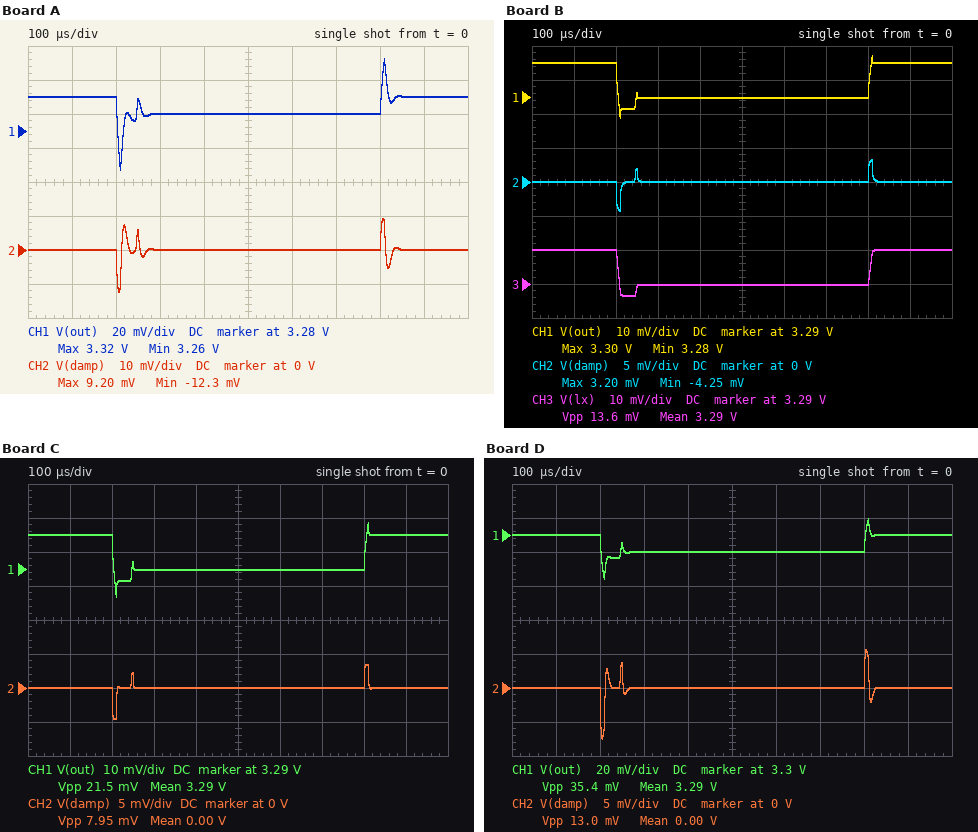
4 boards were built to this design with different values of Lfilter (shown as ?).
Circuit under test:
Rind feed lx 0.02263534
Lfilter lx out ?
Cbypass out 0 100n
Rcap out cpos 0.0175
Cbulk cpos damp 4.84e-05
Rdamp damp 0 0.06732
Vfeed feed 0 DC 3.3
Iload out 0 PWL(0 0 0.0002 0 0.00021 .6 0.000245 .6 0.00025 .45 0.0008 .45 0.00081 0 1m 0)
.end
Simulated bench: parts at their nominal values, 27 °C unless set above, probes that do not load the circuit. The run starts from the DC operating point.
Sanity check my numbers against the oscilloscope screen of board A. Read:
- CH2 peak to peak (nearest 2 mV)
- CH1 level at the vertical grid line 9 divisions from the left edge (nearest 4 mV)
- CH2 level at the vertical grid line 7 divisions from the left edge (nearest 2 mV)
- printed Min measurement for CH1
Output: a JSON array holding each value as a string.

["22 mV", "3.300 V", "0 V", "3.26 V"]
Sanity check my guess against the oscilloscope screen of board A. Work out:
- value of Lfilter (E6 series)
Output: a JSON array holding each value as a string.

["470 nH"]
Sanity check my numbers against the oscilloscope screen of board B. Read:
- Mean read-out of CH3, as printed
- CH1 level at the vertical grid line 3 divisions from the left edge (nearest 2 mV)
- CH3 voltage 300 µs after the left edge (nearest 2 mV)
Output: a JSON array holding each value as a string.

["3.29 V", "3.290 V", "3.290 V"]
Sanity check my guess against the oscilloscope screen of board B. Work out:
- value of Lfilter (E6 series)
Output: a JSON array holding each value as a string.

["68 nH"]
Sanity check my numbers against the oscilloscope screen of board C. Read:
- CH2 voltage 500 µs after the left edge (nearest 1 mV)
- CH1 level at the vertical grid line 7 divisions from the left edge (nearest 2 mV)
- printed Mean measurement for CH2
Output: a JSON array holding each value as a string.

["0 V", "3.290 V", "0.00 V"]
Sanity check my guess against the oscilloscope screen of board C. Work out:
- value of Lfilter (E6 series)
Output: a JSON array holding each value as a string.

["100 nH"]
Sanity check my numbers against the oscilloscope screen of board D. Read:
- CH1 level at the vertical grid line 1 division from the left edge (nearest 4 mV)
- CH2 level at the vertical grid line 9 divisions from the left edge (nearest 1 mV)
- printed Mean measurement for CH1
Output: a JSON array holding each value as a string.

["3.300 V", "0 V", "3.29 V"]
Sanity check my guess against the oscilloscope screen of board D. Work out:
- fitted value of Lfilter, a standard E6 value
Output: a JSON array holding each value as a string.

["220 nH"]
